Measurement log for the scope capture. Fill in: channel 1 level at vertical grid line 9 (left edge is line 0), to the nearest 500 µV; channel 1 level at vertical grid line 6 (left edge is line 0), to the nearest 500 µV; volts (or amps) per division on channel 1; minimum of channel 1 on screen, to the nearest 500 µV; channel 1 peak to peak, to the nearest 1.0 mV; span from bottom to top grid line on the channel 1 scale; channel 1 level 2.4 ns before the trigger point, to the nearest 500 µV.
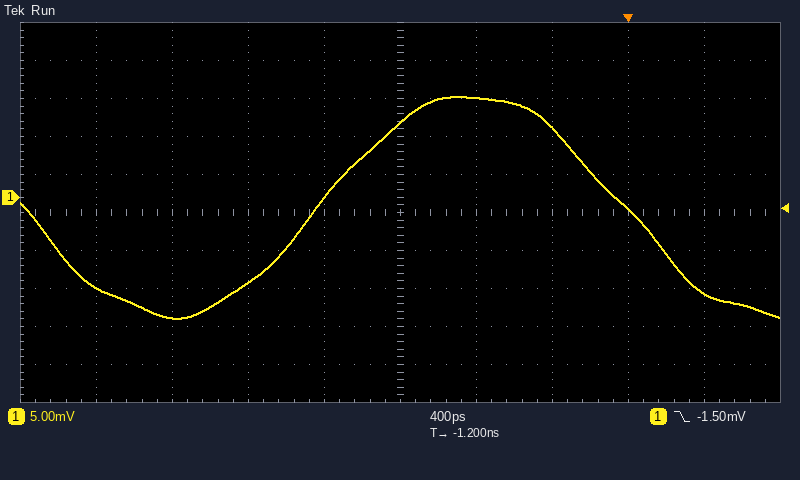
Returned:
-12.5 mV
13.0 mV
5 mV
-16.0 mV
29.0 mV
50 mV
-16.0 mV
